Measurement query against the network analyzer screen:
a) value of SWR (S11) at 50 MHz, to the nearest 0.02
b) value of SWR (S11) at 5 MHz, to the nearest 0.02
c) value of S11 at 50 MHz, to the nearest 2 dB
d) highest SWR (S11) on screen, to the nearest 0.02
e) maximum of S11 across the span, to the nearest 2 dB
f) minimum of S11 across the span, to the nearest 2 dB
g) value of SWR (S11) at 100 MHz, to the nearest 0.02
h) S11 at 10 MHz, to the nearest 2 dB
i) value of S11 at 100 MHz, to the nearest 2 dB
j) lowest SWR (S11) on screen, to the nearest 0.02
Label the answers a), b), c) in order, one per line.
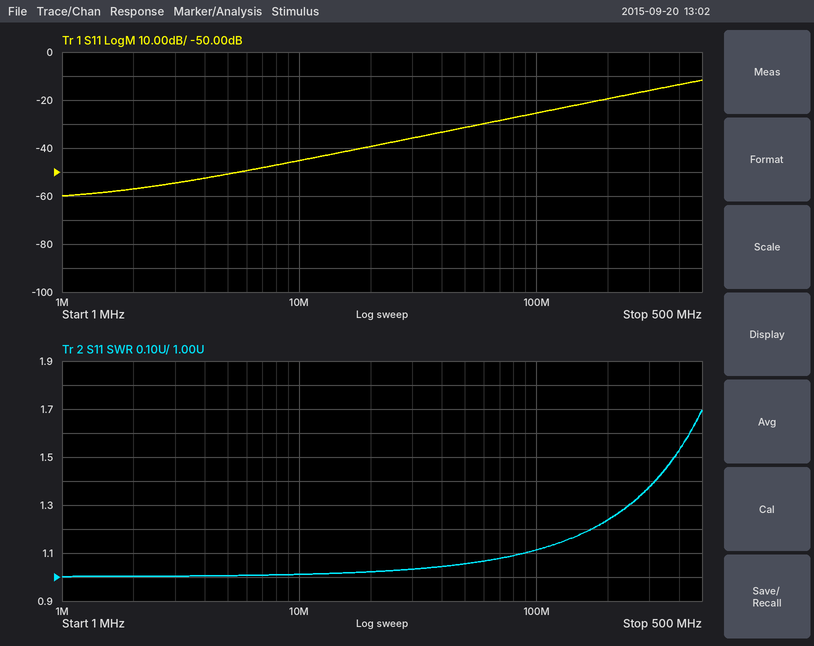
a) 1.06
b) 1.00
c) -32 dB
d) 1.70
e) -12 dB
f) -60 dB
g) 1.12
h) -46 dB
i) -26 dB
j) 1.00
